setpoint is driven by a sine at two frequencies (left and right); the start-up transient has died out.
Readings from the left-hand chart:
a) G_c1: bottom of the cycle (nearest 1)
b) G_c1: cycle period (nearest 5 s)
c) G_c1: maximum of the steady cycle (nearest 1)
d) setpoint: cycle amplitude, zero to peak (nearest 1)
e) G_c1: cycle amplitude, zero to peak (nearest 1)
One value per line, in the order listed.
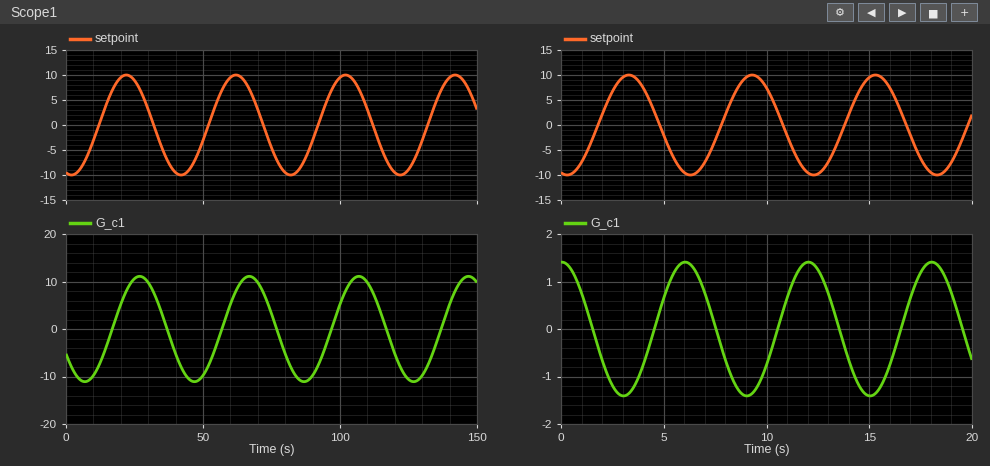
-11
40 s
11
10
11
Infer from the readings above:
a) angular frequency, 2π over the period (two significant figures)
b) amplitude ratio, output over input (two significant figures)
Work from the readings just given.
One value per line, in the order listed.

0.16 rad/s
1.1
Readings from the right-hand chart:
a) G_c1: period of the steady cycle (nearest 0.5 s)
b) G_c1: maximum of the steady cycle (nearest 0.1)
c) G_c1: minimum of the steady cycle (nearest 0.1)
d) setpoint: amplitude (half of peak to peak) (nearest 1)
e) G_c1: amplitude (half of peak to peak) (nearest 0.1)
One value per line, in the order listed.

6.0 s
1.4
-1.4
10
1.4
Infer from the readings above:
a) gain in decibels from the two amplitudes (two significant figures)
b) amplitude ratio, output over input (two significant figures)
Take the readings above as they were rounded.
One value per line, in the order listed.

-17 dB
0.14
